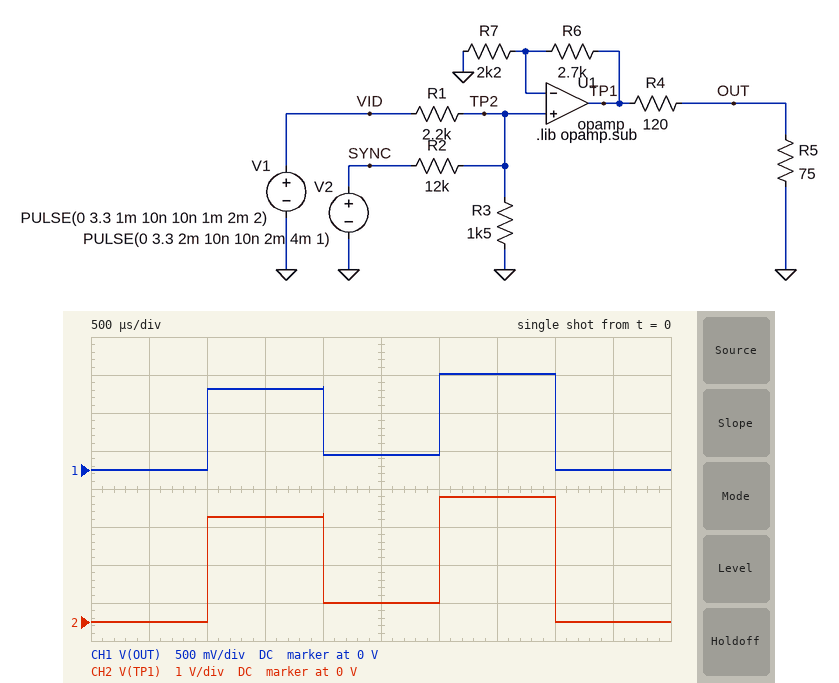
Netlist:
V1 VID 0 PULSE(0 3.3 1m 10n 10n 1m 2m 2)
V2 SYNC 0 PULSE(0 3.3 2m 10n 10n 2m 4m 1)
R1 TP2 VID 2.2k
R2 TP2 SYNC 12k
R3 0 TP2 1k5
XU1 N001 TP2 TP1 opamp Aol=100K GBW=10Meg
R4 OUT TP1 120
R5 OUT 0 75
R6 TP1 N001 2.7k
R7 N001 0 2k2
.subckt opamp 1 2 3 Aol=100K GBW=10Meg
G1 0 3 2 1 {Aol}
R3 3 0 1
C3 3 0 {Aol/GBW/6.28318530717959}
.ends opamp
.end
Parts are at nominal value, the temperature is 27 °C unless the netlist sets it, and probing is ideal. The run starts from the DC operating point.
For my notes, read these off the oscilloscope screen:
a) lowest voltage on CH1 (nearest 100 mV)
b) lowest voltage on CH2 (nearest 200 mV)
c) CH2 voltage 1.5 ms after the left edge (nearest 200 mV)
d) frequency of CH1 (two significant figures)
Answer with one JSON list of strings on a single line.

["0 V", "0 V", "2.8 V", "500 Hz"]
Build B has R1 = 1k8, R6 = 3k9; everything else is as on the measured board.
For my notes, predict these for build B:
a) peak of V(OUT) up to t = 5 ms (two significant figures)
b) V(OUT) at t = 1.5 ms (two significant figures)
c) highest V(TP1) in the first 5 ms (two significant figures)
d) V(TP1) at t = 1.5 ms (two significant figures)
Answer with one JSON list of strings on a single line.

["1.7 V", "1.5 V", "4.5 V", "3.9 V"]
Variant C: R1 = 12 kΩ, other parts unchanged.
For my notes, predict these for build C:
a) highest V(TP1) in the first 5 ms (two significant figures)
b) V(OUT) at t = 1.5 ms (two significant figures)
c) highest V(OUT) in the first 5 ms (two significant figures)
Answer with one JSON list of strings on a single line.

["1.5 V", "280 mV", "570 mV"]
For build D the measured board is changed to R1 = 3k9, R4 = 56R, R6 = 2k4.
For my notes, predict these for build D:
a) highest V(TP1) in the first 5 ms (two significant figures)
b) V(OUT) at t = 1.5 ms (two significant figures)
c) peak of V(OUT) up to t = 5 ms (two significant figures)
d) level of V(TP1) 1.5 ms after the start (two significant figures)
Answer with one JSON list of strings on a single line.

["2.3 V", "1.0 V", "1.3 V", "1.8 V"]
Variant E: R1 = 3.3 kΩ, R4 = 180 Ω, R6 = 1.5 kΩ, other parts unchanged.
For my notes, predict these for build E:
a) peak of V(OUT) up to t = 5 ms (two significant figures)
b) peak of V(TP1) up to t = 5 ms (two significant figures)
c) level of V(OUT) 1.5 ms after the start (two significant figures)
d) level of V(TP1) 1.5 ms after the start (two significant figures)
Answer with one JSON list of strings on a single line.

["600 mV", "2.0 V", "470 mV", "1.6 V"]
